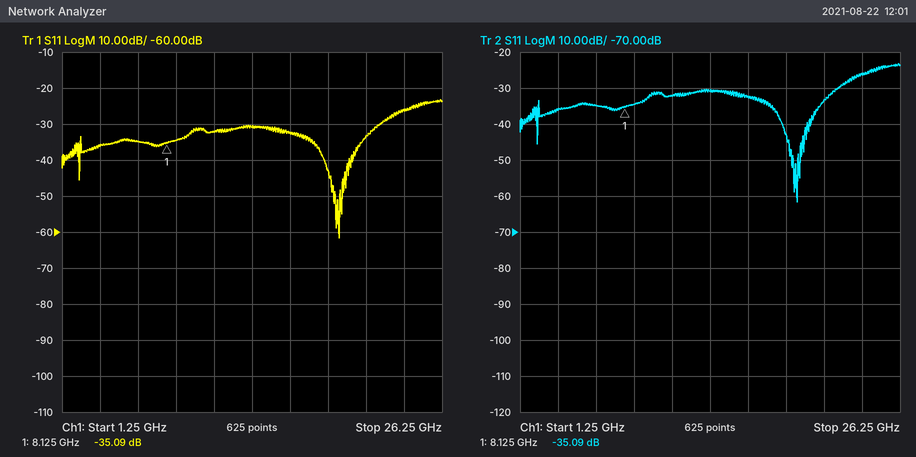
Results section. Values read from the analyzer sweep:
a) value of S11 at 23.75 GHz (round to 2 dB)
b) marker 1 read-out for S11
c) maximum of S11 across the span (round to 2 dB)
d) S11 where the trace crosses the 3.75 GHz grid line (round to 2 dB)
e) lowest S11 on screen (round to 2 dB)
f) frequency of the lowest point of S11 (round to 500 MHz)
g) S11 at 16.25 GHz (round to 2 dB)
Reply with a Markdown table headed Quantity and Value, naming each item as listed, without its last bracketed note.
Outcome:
| Quantity | Value |
|---|---|
| value of S11 at 23.75 GHz | -26 dB |
| marker 1 read-out for S11 | -35.09 dB |
| maximum of S11 across the span | -24 dB |
| S11 where the trace crosses the 3.75 GHz grid line | -36 dB |
| lowest S11 on screen | -62 dB |
| frequency of the lowest point of S11 | 19.5 GHz |
| S11 at 16.25 GHz | -32 dB |
